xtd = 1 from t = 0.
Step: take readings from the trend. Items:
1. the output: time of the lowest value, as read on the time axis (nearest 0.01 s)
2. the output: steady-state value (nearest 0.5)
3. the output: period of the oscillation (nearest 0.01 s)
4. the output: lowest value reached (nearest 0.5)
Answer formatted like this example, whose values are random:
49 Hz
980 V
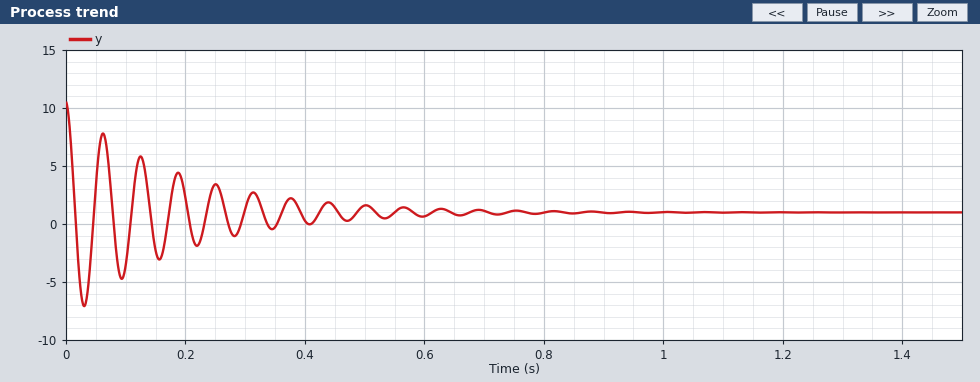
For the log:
0.03 s
1.0
0.06 s
-7.0
